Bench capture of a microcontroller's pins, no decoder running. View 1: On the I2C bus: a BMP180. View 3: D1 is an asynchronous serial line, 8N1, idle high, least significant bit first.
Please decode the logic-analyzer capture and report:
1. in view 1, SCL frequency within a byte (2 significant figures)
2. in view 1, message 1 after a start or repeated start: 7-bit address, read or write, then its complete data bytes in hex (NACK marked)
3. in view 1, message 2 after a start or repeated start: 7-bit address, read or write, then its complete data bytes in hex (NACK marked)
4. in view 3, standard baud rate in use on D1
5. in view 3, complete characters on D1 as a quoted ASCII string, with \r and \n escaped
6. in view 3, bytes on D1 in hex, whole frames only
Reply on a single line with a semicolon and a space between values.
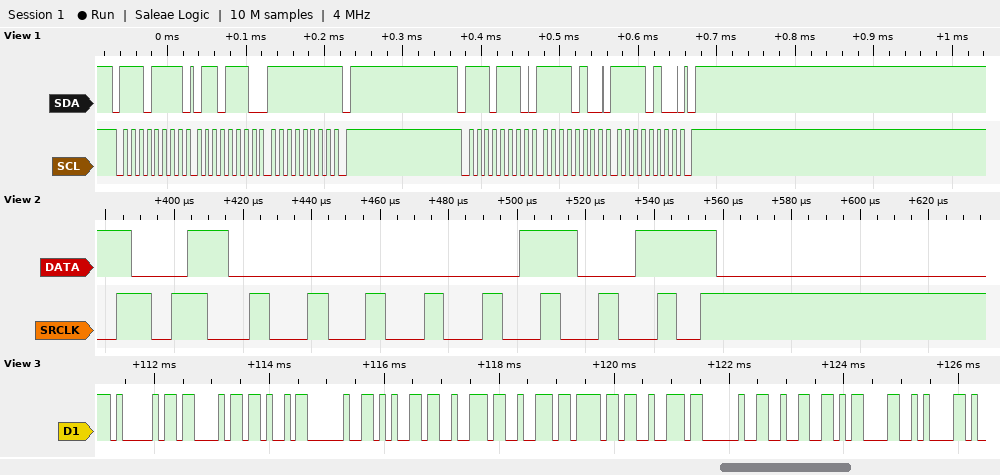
100 kHz; 0x77 read: 6E FF NACK; 0x77 write: F4 F4; 9600 baud; "ACK error 2\r\n"; 41 43 4B 20 65 72 72 6F 72 20 32 0D 0A
